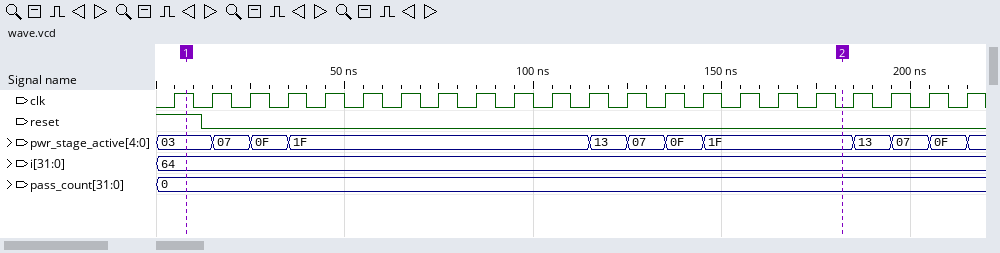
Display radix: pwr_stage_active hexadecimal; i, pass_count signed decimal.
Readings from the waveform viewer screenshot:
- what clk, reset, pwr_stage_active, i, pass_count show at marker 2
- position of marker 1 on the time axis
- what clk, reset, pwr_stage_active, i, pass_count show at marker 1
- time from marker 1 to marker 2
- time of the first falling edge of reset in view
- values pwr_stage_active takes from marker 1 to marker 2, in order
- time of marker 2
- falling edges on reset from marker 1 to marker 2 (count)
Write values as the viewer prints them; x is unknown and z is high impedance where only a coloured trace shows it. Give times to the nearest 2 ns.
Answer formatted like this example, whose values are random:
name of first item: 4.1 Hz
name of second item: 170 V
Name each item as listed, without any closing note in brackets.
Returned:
what clk, reset, pwr_stage_active, i, pass_count show at marker 2: clk=0, reset=0, pwr_stage_active=1F, i=64, pass_count=0
position of marker 1 on the time axis: 8 ns
what clk, reset, pwr_stage_active, i, pass_count show at marker 1: clk=1, reset=1, pwr_stage_active=03, i=64, pass_count=0
time from marker 1 to marker 2: 174 ns
time of the first falling edge of reset in view: 12 ns
values pwr_stage_active takes from marker 1 to marker 2, in order: 03, 07, 0F, 1F, 13, 07, 0F, 1F
time of marker 2: 182 ns
falling edges on reset from marker 1 to marker 2: 1
